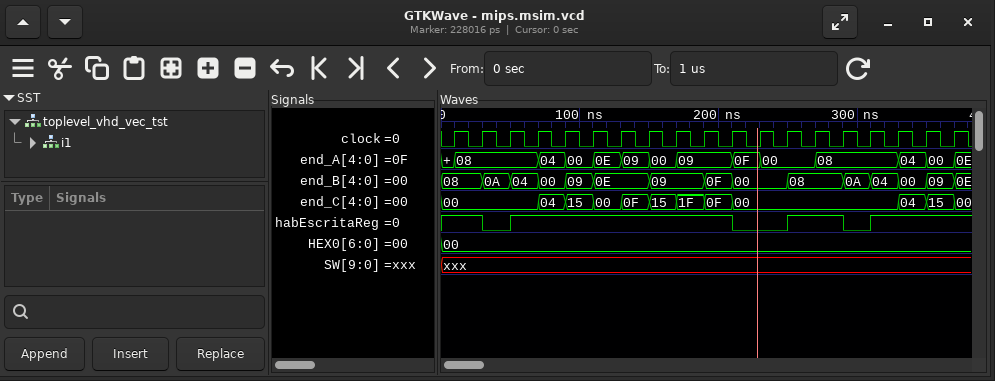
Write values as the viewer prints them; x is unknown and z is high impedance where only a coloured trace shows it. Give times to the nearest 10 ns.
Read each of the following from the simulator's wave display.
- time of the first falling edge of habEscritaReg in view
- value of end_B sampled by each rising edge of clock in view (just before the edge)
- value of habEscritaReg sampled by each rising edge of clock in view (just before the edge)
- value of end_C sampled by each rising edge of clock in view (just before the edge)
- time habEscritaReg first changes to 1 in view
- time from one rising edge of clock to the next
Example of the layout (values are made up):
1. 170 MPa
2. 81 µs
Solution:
1. 30 ns
2. 08, 08, 0A, 04, 00, 09, 0E, 0E, 09, 09, 0F, 00, 00, 08, 08, 0A, 04, 00, 09
3. 1 1 0 1 1 1 1 1 1 1 1 0 0 1 1 0 1 1 1
4. 00, 00, 00, 00, 04, 15, 00, 0F, 15, 1F, 0F, 00, 00, 00, 00, 00, 00, 04, 15
5. 50 ns
6. 20 ns
